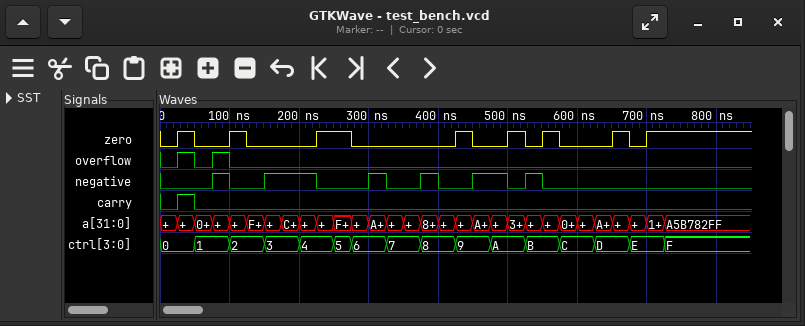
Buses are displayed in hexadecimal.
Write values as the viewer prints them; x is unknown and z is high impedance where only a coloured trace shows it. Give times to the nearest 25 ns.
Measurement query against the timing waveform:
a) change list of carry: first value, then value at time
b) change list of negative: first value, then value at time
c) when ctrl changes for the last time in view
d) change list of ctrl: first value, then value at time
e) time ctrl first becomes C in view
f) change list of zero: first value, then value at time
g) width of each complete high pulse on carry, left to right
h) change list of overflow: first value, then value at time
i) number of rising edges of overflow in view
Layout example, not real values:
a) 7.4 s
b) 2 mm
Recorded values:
a) 0, 1 at 25 ns, 0 at 50 ns
b) 0, 1 at 75 ns, 0 at 100 ns, 1 at 150 ns, 0 at 225 ns, 1 at 300 ns, 0 at 325 ns, 1 at 375 ns, 0 at 400 ns, 1 at 450 ns, 0 at 500 ns, 1 at 525 ns, 0 at 550 ns
c) 725 ns
d) 0, 1 at 50 ns, 2 at 100 ns, 3 at 150 ns, 4 at 200 ns, 5 at 250 ns, 6 at 275 ns, 7 at 325 ns, 8 at 375 ns, 9 at 425 ns, A at 475 ns, B at 525 ns, C at 575 ns, D at 625 ns, E at 675 ns, F at 725 ns
e) 575 ns
f) 0, 1 at 25 ns, 0 at 50 ns, 1 at 100 ns, 0 at 125 ns, 1 at 225 ns, 0 at 275 ns, 1 at 425 ns, 0 at 450 ns, 1 at 500 ns, 0 at 525 ns, 1 at 550 ns, 0 at 575 ns, 1 at 650 ns, 0 at 675 ns, 1 at 700 ns
g) 25 ns
h) 0, 1 at 25 ns, 0 at 50 ns, 1 at 75 ns, 0 at 100 ns
i) 2
